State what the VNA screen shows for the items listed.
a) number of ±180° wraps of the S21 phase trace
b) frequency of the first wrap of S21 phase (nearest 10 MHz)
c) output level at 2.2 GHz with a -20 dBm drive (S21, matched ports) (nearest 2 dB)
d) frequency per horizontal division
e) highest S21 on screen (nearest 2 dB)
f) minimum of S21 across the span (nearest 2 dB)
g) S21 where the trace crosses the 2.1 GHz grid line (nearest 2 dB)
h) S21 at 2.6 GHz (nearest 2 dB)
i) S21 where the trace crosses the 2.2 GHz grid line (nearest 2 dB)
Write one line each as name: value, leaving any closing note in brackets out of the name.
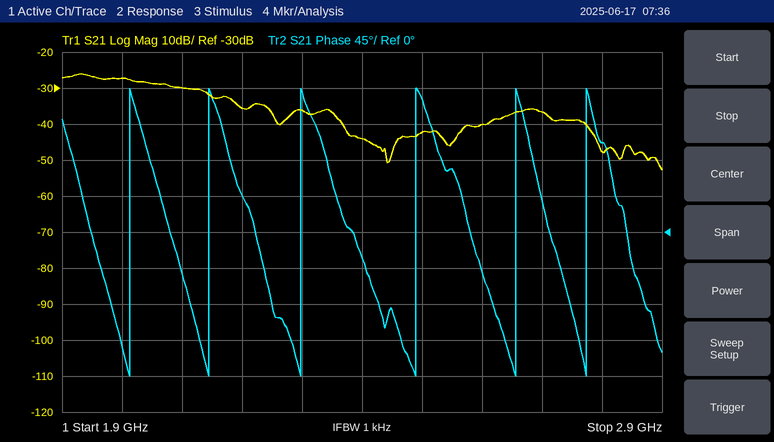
number of ±180° wraps of the S21 phase trace: 6
frequency of the first wrap of S21 phase: 2.01 GHz
output level at 2.2 GHz with a -20 dBm drive (S21, matched ports): -56 dBm
frequency per horizontal division: 100 MHz
highest S21 on screen: -26 dB
minimum of S21 across the span: -52 dB
S21 where the trace crosses the 2.1 GHz grid line: -30 dB
S21 at 2.6 GHz: -40 dB
S21 where the trace crosses the 2.2 GHz grid line: -36 dB
